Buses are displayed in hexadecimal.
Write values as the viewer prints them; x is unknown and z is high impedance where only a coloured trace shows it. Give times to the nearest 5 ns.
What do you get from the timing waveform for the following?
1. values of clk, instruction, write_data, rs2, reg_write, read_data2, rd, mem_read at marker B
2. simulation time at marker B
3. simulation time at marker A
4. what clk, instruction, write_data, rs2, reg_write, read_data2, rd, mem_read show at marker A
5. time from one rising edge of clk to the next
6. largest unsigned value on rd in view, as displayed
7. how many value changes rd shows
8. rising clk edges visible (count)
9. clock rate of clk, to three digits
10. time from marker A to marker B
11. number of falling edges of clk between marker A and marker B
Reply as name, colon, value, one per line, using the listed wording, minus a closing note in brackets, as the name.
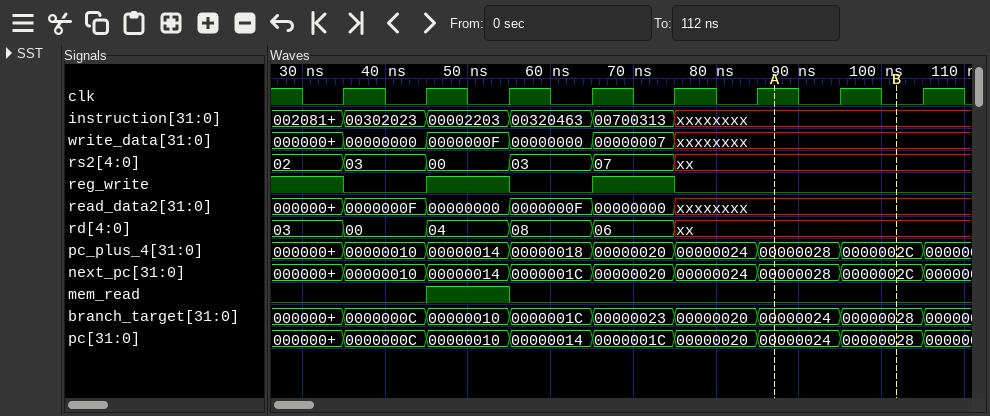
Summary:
values of clk, instruction, write_data, rs2, reg_write, read_data2, rd, mem_read at marker B: clk=0, instruction=xxxxxxxx, write_data=xxxxxxxx, rs2=xx, reg_write=0, read_data2=xxxxxxxx, rd=xx, mem_read=0
simulation time at marker B: 100 ns
simulation time at marker A: 85 ns
what clk, instruction, write_data, rs2, reg_write, read_data2, rd, mem_read show at marker A: clk=1, instruction=xxxxxxxx, write_data=xxxxxxxx, rs2=xx, reg_write=0, read_data2=xxxxxxxx, rd=xx, mem_read=0
time from one rising edge of clk to the next: 10 ns
largest unsigned value on rd in view, as displayed: 08
how many value changes rd shows: 5
rising clk edges visible: 8
clock rate of clk, to three digits: 100 MHz
time from marker A to marker B: 15 ns
number of falling edges of clk between marker A and marker B: 2
